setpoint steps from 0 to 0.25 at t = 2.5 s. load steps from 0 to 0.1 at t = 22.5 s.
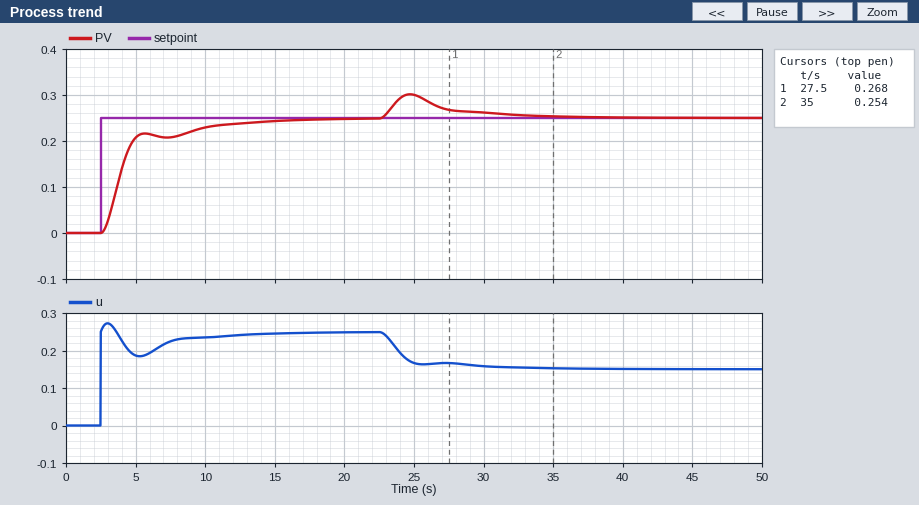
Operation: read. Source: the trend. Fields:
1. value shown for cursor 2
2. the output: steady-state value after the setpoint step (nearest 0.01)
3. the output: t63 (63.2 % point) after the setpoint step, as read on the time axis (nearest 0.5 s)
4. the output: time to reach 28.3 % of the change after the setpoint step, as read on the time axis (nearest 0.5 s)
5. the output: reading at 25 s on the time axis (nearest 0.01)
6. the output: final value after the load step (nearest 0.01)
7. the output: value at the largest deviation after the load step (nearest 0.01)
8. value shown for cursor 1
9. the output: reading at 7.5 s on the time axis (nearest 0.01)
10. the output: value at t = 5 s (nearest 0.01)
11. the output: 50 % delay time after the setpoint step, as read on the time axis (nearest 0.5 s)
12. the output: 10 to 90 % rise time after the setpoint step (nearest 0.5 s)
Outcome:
0.254
0.25
4.0 s
3.5 s
0.30
0.25
0.30
0.268
0.21
0.21
4.0 s
6.5 s
